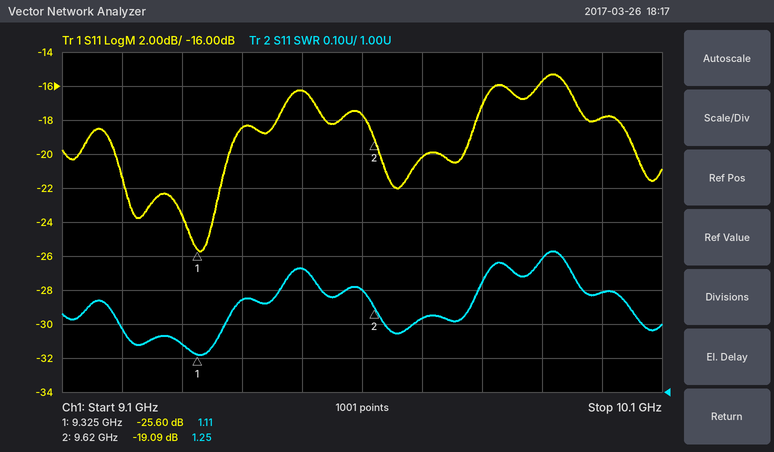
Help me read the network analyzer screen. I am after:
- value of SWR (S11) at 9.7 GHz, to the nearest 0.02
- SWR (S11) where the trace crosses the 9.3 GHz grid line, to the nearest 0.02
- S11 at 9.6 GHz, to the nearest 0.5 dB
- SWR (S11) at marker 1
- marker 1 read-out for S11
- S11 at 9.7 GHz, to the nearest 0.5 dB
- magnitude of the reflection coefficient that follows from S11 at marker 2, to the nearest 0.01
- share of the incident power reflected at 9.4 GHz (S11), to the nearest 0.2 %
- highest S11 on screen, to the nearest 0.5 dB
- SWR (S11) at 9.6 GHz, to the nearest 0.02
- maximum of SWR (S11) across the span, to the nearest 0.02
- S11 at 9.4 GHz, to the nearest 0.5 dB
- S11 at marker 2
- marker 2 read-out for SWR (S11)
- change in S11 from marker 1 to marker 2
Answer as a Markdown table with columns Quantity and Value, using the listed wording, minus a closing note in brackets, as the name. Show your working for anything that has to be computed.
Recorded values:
| Quantity | Value |
|---|---|
| value of SWR (S11) at 9.7 GHz, to the nearest 0.02 | 1.22 |
| SWR (S11) where the trace crosses the 9.3 GHz grid line, to the nearest 0.02 | 1.14 |
| S11 at 9.6 GHz, to the nearest 0.5 dB | -17.5 dB |
| SWR (S11) at marker 1 | 1.11 |
| marker 1 read-out for S11 | -25.60 dB |
| S11 at 9.7 GHz, to the nearest 0.5 dB | -20.0 dB |
| magnitude of the reflection coefficient that follows from S11 at marker 2, to the nearest 0.01 | 10^(-19.09/20) ≈ 0.11 |
| share of the incident power reflected at 9.4 GHz (S11), to the nearest 0.2 % | 10^(-18.5/10) ≈ 1.4 % |
| highest S11 on screen, to the nearest 0.5 dB | -15.5 dB |
| SWR (S11) at 9.6 GHz, to the nearest 0.02 | 1.30 |
| maximum of SWR (S11) across the span, to the nearest 0.02 | 1.42 |
| S11 at 9.4 GHz, to the nearest 0.5 dB | -18.5 dB |
| S11 at marker 2 | -19.09 dB |
| marker 2 read-out for SWR | 1.25 |
| change in S11 from marker 1 to marker 2 | -19.09 − (-25.6) = 6.51 dB |
